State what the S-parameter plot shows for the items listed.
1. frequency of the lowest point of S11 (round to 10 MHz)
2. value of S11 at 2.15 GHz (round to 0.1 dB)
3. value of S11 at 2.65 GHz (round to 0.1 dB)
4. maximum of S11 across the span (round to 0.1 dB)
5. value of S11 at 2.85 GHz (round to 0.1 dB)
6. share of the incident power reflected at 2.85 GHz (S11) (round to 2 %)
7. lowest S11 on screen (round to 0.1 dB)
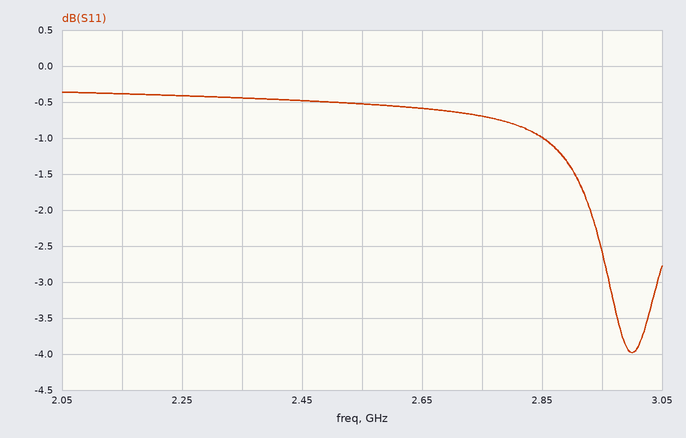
3.00 GHz
-0.4 dB
-0.6 dB
-0.4 dB
-1.0 dB
80 %
-4.0 dB
